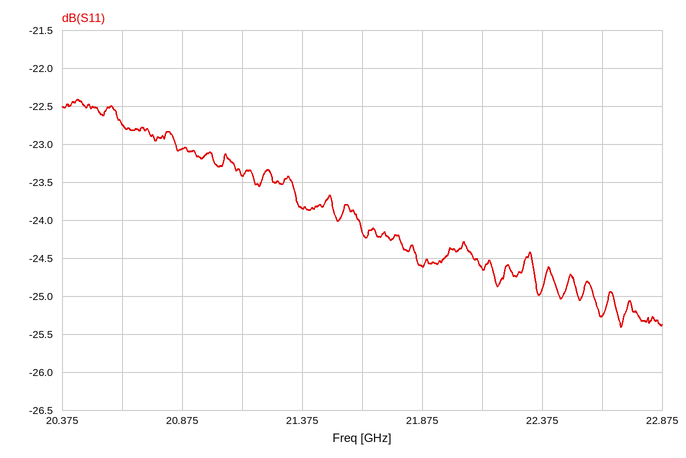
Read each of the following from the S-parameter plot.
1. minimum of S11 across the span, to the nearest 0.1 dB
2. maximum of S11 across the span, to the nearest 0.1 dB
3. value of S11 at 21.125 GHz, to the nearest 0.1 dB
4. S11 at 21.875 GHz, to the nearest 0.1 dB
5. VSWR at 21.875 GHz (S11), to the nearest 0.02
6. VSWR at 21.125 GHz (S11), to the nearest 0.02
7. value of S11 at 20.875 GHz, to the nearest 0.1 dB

-25.4 dB
-22.4 dB
-23.4 dB
-24.6 dB
1.12
1.14
-23.1 dB
